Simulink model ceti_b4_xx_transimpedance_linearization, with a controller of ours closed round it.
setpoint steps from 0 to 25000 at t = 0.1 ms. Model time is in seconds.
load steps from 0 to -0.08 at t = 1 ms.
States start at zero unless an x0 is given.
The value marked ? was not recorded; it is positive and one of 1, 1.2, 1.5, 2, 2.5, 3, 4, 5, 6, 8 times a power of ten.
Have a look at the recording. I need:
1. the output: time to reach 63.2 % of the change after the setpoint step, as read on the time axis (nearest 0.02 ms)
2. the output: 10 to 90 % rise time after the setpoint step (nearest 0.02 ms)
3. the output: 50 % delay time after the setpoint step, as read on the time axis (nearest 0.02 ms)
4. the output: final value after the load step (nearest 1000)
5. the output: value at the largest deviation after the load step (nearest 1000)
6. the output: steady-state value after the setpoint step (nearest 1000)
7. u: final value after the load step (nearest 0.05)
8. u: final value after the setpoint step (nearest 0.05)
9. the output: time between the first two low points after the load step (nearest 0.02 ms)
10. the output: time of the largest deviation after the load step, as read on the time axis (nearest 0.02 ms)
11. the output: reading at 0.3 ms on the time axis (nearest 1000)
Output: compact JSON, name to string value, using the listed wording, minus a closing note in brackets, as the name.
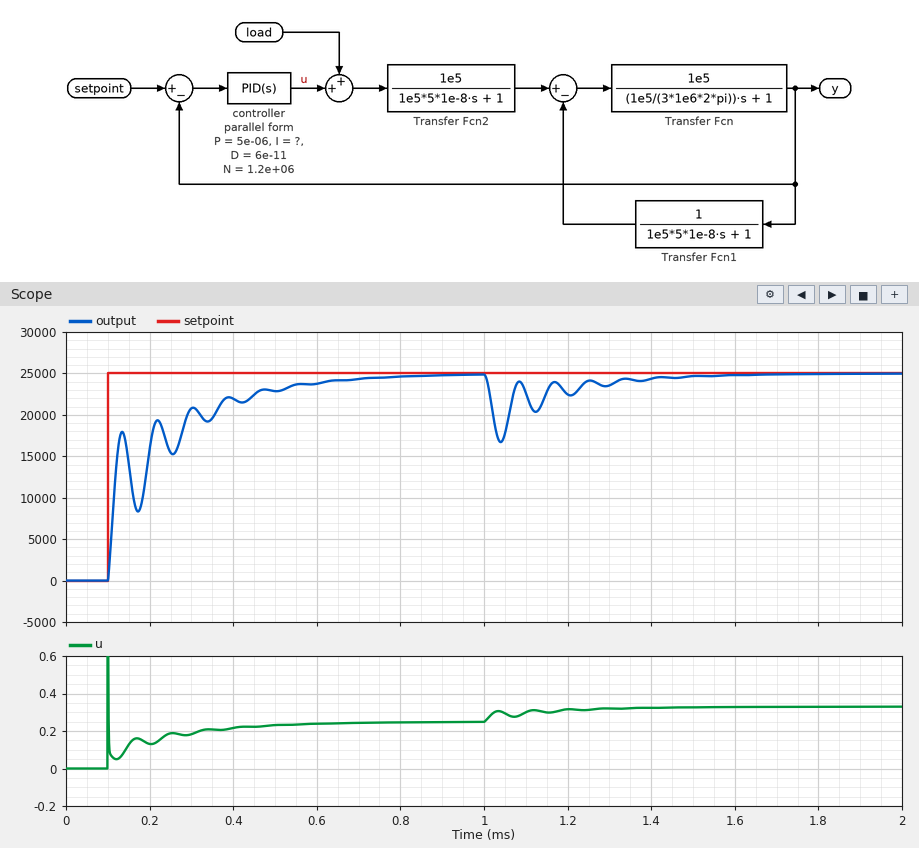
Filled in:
{"the output: time to reach 63.2 % of the change after the setpoint step, as read on the time axis": "0.12 ms", "the output: 10 to 90 % rise time after the setpoint step": "0.34 ms", "the output: 50 % delay time after the setpoint step, as read on the time axis": "0.12 ms", "the output: final value after the load step": "25000", "the output: value at the largest deviation after the load step": "17000", "the output: steady-state value after the setpoint step": "25000", "u: final value after the load step": "0.35", "u: final value after the setpoint step": "0.25", "the output: time between the first two low points after the load step": "0.08 ms", "the output: time of the largest deviation after the load step, as read on the time axis": "1.04 ms", "the output: reading at 0.3 ms on the time axis": "21000"}
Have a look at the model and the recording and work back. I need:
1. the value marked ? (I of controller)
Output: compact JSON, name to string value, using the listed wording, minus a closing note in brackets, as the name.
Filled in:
{"the value marked ?": "0.08"}
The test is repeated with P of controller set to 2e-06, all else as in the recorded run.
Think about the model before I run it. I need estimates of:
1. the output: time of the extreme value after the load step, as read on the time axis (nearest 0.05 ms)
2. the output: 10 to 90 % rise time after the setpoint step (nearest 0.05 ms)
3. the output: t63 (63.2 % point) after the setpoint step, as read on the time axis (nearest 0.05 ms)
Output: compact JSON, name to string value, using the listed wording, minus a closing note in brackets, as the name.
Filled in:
{"the output: time of the extreme value after the load step, as read on the time axis": "1.05 ms", "the output: 10 to 90 % rise time after the setpoint step": "0.30 ms", "the output: t63 (63.2 % point) after the setpoint step, as read on the time axis": "0.20 ms"}
